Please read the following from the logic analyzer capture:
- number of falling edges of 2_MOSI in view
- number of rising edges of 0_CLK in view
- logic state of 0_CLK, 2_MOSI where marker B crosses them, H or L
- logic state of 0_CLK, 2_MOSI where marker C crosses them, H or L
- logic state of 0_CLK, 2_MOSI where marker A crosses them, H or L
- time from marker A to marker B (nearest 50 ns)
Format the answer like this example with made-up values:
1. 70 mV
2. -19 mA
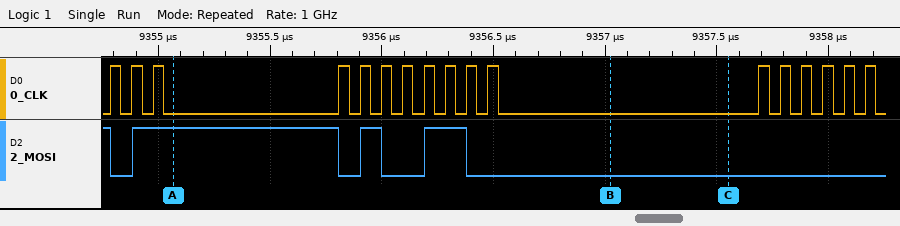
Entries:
1. 4
2. 17
3. 0_CLK=L, 2_MOSI=L
4. 0_CLK=L, 2_MOSI=L
5. 0_CLK=L, 2_MOSI=H
6. 1950 ns
